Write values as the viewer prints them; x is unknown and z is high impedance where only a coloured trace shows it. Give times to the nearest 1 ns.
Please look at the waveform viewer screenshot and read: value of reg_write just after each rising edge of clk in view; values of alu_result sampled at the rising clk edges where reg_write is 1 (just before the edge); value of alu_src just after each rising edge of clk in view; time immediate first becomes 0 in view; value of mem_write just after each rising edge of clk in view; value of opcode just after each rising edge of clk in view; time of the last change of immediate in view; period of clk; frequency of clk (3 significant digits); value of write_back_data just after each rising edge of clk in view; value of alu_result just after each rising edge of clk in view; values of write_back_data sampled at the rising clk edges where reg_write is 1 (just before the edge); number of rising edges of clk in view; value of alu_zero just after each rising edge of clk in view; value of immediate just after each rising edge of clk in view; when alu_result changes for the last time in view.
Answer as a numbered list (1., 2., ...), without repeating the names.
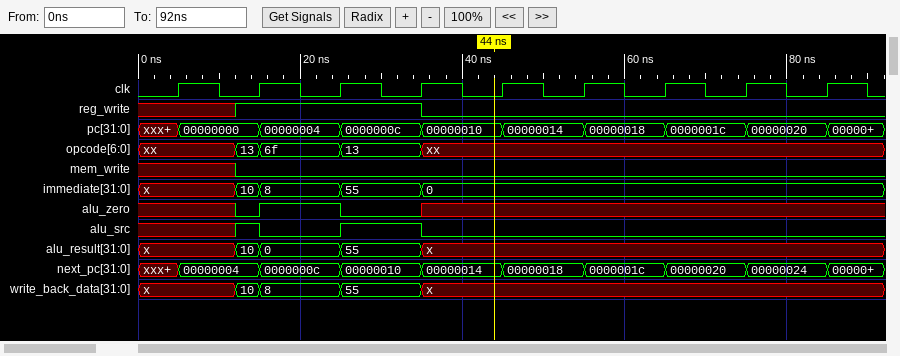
1. x 1 1 0 0 0 0 0 0
2. 10, 0, 55
3. x 0 1 0 0 0 0 0 0
4. 35 ns
5. x 0 0 0 0 0 0 0 0
6. xx, 6f, 13, xx, xx, xx, xx, xx, xx
7. 35 ns
8. 10 ns
9. 100 MHz
10. x, 8, 55, x, x, x, x, x, x
11. x, 0, 55, x, x, x, x, x, x
12. 10, 8, 55
13. 9
14. x 1 0 x x x x x x
15. x, 8, 55, 0, 0, 0, 0, 0, 0
16. 35 ns
